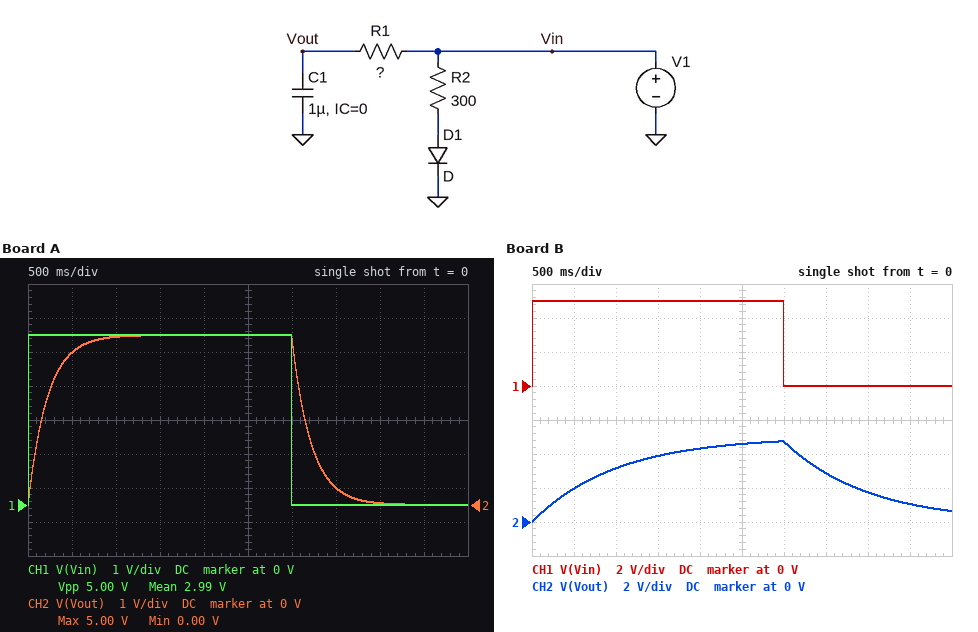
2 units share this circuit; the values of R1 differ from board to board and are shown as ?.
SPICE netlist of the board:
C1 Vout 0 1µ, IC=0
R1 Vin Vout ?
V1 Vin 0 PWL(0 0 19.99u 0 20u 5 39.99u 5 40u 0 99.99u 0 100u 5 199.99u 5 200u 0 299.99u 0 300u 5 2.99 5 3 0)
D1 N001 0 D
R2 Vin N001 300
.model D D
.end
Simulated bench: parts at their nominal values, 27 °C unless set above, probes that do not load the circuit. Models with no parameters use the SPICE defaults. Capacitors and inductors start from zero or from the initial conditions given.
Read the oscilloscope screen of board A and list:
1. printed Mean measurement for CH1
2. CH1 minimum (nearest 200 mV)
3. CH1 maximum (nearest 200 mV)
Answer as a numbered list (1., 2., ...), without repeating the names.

1. 2.99 V
2. 0 V
3. 5.0 V
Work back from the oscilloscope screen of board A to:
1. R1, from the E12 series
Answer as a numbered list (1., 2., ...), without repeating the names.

1. 220 kΩ
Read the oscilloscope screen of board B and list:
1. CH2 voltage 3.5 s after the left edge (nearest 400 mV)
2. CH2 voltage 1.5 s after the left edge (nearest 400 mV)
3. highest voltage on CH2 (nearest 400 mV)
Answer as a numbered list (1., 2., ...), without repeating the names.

1. 2.8 V
2. 4.0 V
3. 4.8 V
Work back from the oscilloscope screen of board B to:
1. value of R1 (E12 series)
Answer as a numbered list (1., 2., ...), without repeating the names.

1. 1 MΩ
